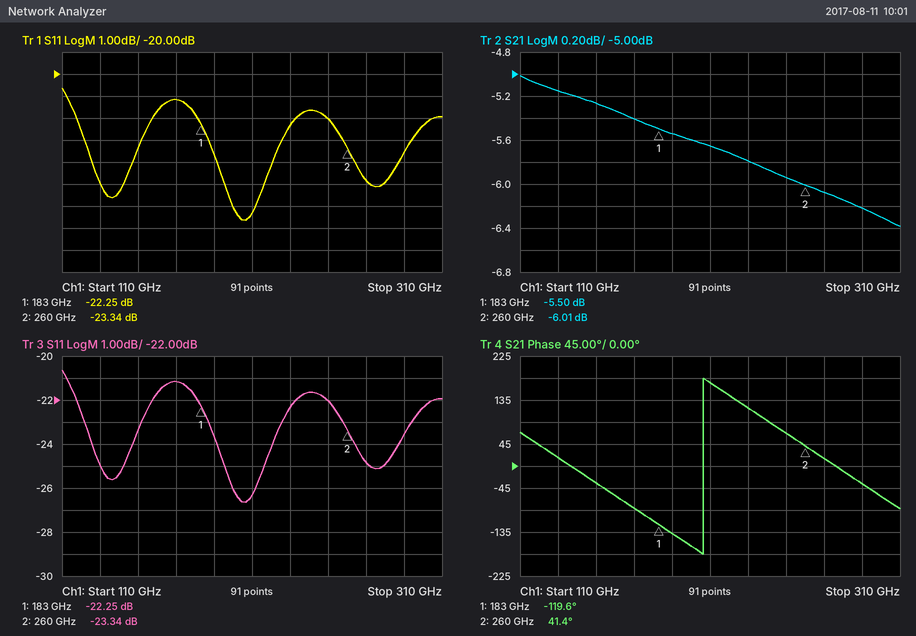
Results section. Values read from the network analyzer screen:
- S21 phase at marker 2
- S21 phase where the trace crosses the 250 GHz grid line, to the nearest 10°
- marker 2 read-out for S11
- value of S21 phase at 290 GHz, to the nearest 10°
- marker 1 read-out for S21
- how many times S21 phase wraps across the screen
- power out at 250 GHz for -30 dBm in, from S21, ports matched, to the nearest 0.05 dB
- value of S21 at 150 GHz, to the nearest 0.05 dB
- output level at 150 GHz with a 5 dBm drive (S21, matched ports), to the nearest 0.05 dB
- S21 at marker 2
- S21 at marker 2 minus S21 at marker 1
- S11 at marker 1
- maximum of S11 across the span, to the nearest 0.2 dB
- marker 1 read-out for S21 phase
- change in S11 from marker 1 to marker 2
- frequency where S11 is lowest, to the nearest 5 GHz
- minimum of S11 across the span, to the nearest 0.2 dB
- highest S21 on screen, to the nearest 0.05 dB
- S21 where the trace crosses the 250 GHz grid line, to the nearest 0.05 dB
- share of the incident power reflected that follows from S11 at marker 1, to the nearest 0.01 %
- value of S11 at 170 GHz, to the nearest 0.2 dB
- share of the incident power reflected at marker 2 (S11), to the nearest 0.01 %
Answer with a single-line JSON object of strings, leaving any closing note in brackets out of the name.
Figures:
{"S21 phase at marker 2": "41.4°", "S21 phase where the trace crosses the 250 GHz grid line, to the nearest 10°": "70°", "marker 2 read-out for S11": "-23.34 dB", "value of S21 phase at 290 GHz, to the nearest 10°": "-40°", "marker 1 read-out for S21": "-5.50 dB", "how many times S21 phase wraps across the screen": "1", "power out at 250 GHz for -30 dBm in, from S21, ports matched, to the nearest 0.05 dB": "-35.95 dBm", "value of S21 at 150 GHz, to the nearest 0.05 dB": "-5.25 dB", "output level at 150 GHz with a 5 dBm drive (S21, matched ports), to the nearest 0.05 dB": "-0.25 dBm", "S21 at marker 2": "-6.01 dB", "S21 at marker 2 minus S21 at marker 1": "-0.51 dB", "S11 at marker 1": "-22.25 dB", "maximum of S11 across the span, to the nearest 0.2 dB": "-20.6 dB", "marker 1 read-out for S21 phase": "-119.6°", "change in S11 from marker 1 to marker 2": "-1.09 dB", "frequency where S11 is lowest, to the nearest 5 GHz": "205 GHz", "minimum of S11 across the span, to the nearest 0.2 dB": "-26.6 dB", "highest S21 on screen, to the nearest 0.05 dB": "-5.00 dB", "S21 where the trace crosses the 250 GHz grid line, to the nearest 0.05 dB": "-5.95 dB", "share of the incident power reflected that follows from S11 at marker 1, to the nearest 0.01 %": "0.60 %", "value of S11 at 170 GHz, to the nearest 0.2 dB": "-21.2 dB", "share of the incident power reflected at marker 2 (S11), to the nearest 0.01 %": "0.46 %"}
